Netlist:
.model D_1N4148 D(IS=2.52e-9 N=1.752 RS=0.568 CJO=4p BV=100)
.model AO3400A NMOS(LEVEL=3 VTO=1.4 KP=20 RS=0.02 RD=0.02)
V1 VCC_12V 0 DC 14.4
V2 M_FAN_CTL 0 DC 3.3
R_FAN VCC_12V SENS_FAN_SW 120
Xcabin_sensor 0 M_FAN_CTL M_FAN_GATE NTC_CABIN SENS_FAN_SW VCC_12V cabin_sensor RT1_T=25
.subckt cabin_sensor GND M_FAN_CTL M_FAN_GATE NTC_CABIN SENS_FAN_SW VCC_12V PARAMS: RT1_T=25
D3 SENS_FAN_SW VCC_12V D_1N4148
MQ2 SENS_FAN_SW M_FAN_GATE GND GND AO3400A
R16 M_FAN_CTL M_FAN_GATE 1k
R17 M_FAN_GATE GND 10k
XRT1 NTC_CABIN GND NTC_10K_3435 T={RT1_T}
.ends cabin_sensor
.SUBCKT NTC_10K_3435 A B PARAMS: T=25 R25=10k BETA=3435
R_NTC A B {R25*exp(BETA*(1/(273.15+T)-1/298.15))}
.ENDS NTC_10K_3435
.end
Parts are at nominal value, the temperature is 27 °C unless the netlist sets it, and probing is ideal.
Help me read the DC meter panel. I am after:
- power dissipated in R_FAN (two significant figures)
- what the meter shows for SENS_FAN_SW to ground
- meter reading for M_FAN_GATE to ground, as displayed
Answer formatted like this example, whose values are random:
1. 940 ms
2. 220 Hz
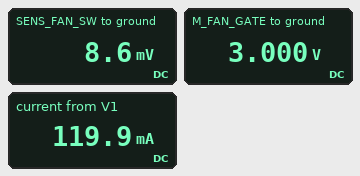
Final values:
1. 1.7 W
2. 8.6 mV
3. 3.000 V
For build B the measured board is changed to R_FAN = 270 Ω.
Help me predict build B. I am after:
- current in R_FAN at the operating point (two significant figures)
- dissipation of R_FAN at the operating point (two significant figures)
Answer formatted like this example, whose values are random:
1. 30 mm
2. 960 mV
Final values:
1. 53 mA
2. 770 mW
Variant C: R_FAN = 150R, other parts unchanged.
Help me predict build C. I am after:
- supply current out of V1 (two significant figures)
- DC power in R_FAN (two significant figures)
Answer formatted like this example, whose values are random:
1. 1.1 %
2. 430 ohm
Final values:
1. 96 mA
2. 1.4 W
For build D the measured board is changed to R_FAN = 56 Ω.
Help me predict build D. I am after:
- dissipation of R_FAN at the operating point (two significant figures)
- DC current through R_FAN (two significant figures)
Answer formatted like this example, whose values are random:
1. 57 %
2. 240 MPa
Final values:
1. 3.7 W
2. 260 mA
